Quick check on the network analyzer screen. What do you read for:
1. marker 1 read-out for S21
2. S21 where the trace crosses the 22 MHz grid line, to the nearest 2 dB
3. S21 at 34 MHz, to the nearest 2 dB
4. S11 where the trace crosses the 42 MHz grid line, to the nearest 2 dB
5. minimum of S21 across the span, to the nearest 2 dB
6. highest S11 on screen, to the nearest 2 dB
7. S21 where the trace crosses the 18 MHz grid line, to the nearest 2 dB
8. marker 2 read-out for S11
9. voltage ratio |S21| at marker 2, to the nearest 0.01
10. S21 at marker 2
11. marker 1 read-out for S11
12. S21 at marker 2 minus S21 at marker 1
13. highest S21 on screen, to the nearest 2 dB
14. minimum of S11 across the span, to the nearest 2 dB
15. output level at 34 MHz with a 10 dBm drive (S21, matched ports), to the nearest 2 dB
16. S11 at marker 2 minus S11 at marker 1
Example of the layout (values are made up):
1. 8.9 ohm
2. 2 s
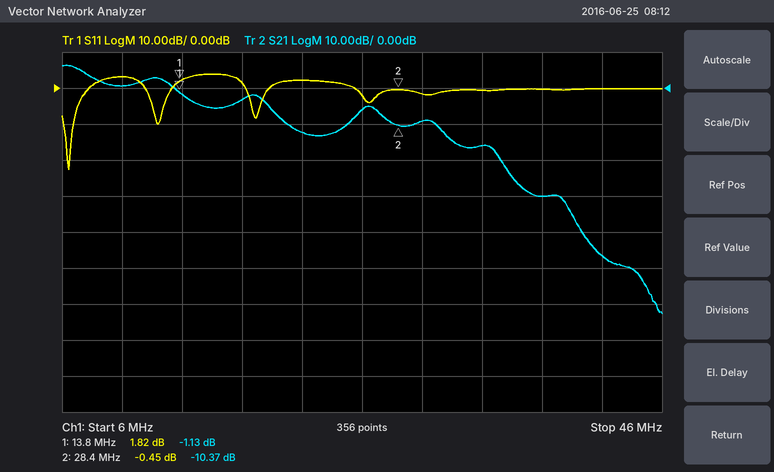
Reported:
1. -1.13 dB
2. -12 dB
3. -16 dB
4. 0 dB
5. -62 dB
6. 4 dB
7. -4 dB
8. -0.45 dB
9. 0.30
10. -10.37 dB
11. 1.82 dB
12. -9.24 dB
13. 6 dB
14. -22 dB
15. -6 dBm
16. -2.27 dB
